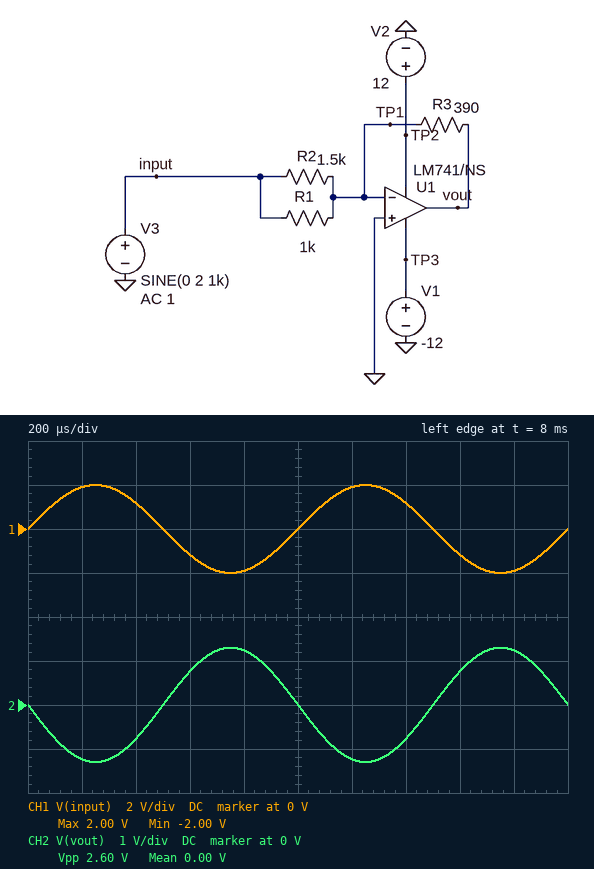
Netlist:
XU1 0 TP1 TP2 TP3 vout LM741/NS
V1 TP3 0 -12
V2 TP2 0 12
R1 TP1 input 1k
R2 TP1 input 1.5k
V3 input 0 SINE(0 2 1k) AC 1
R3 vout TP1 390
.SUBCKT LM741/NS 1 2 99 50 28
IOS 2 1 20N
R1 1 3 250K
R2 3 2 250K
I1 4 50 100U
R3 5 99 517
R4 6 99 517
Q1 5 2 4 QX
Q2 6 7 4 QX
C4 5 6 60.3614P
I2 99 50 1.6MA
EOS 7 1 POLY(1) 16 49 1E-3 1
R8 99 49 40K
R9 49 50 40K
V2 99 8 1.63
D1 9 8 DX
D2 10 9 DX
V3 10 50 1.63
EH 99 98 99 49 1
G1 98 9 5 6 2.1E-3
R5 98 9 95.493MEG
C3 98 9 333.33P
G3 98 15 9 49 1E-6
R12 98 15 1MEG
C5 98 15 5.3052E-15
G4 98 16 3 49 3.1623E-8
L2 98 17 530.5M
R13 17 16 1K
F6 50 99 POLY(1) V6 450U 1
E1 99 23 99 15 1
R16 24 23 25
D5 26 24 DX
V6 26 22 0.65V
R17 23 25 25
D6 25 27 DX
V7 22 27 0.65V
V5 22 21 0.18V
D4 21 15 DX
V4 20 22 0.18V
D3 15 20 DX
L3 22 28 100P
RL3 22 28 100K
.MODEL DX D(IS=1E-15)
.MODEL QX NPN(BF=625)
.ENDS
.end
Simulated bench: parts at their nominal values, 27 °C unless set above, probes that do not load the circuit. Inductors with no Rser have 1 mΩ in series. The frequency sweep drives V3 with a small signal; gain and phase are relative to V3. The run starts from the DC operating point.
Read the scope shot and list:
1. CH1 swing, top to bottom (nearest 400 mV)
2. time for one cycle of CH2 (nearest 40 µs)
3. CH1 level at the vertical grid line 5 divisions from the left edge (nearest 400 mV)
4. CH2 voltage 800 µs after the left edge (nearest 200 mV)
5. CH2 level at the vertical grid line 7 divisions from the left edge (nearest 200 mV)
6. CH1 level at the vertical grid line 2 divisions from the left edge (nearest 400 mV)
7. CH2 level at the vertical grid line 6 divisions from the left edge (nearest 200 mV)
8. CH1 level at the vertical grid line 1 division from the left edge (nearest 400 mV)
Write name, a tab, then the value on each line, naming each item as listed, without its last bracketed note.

CH1 swing, top to bottom	4.0 V
time for one cycle of CH2	1.00 ms
CH1 level at the vertical grid line 5 divisions from the left edge	0 V
CH2 voltage 800 µs after the left edge	1.2 V
CH2 level at the vertical grid line 7 divisions from the left edge	-800 mV
CH1 level at the vertical grid line 2 divisions from the left edge	1.2 V
CH2 level at the vertical grid line 6 divisions from the left edge	-1.2 V
CH1 level at the vertical grid line 1 division from the left edge	2.0 V
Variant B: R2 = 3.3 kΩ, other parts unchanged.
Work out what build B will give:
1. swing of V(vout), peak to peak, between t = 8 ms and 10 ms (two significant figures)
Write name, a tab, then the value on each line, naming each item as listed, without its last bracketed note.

swing of V(vout), peak to peak, between t = 8 ms and 10 ms	2.0 V
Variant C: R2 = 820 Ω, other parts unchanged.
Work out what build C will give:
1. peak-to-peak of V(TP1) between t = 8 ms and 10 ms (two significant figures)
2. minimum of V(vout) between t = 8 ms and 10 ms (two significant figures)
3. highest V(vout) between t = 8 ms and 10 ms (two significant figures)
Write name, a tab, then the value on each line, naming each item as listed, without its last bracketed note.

peak-to-peak of V(TP1) between t = 8 ms and 10 ms	5.1 mV
minimum of V(vout) between t = 8 ms and 10 ms	-1.7 V
highest V(vout) between t = 8 ms and 10 ms	1.7 V
